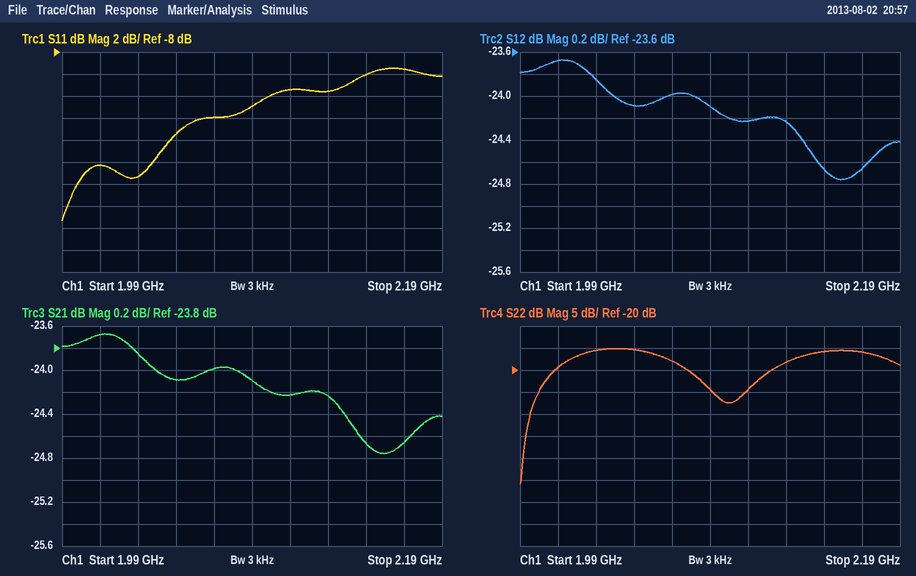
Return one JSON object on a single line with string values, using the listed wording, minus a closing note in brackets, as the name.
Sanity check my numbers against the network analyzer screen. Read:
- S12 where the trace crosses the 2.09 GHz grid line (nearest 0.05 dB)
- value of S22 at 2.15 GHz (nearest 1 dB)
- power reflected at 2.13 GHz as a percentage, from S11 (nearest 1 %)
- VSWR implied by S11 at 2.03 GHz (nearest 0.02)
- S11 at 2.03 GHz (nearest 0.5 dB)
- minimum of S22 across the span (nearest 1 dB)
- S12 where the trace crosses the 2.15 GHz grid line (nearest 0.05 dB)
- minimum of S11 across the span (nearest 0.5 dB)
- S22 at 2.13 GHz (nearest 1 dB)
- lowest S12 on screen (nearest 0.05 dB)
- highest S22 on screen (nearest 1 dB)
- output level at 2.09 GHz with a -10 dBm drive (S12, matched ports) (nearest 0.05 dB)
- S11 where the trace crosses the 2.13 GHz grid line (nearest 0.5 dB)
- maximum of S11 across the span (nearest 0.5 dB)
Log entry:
{"S12 where the trace crosses the 2.09 GHz grid line": "-24.10 dB", "value of S22 at 2.15 GHz": "-16 dB", "power reflected at 2.13 GHz as a percentage, from S11": "7 %", "VSWR implied by S11 at 2.03 GHz": "1.24", "S11 at 2.03 GHz": "-19.5 dB", "minimum of S22 across the span": "-46 dB", "S12 where the trace crosses the 2.15 GHz grid line": "-24.65 dB", "minimum of S11 across the span": "-23.5 dB", "S22 at 2.13 GHz": "-18 dB", "lowest S12 on screen": "-24.75 dB", "highest S22 on screen": "-15 dB", "output level at 2.09 GHz with a -10 dBm drive (S12, matched ports)": "-34.10 dBm", "S11 where the trace crosses the 2.13 GHz grid line": "-11.5 dB", "maximum of S11 across the span": "-9.5 dB"}
